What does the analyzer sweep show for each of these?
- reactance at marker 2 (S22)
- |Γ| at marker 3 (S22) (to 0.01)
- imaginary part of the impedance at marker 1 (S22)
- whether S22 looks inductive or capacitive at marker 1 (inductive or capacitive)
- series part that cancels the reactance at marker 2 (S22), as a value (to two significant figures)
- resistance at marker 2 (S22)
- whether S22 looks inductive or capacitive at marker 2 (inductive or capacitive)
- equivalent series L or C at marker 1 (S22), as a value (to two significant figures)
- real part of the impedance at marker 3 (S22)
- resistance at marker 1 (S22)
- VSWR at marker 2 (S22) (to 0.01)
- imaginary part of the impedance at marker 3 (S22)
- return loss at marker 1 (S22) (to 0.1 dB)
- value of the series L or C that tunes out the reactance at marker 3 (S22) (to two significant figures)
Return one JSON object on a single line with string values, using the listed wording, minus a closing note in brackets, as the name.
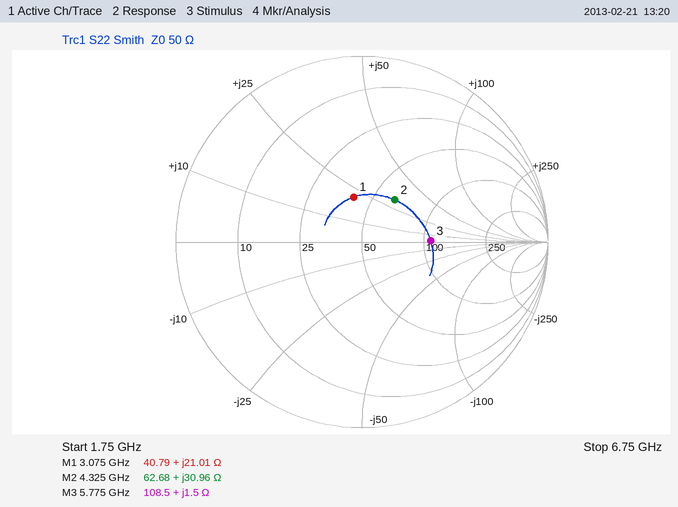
{"reactance at marker 2": "+30.96 Ω", "|Γ| at marker 3 (S22)": "0.37", "imaginary part of the impedance at marker 1": "+21.01 Ω", "whether S22 looks inductive or capacitive at marker 1": "inductive", "series part that cancels the reactance at marker 2 (S22), as a value": "1.2 pF", "resistance at marker 2": "62.68 Ω", "whether S22 looks inductive or capacitive at marker 2": "inductive", "equivalent series L or C at marker 1 (S22), as a value": "1.1 nH", "real part of the impedance at marker 3": "108.5 Ω", "resistance at marker 1": "40.79 Ω", "VSWR at marker 2 (S22)": "1.80", "imaginary part of the impedance at marker 3": "+1.5 Ω", "return loss at marker 1 (S22)": "12.2 dB", "value of the series L or C that tunes out the reactance at marker 3 (S22)": "18 pF"}
